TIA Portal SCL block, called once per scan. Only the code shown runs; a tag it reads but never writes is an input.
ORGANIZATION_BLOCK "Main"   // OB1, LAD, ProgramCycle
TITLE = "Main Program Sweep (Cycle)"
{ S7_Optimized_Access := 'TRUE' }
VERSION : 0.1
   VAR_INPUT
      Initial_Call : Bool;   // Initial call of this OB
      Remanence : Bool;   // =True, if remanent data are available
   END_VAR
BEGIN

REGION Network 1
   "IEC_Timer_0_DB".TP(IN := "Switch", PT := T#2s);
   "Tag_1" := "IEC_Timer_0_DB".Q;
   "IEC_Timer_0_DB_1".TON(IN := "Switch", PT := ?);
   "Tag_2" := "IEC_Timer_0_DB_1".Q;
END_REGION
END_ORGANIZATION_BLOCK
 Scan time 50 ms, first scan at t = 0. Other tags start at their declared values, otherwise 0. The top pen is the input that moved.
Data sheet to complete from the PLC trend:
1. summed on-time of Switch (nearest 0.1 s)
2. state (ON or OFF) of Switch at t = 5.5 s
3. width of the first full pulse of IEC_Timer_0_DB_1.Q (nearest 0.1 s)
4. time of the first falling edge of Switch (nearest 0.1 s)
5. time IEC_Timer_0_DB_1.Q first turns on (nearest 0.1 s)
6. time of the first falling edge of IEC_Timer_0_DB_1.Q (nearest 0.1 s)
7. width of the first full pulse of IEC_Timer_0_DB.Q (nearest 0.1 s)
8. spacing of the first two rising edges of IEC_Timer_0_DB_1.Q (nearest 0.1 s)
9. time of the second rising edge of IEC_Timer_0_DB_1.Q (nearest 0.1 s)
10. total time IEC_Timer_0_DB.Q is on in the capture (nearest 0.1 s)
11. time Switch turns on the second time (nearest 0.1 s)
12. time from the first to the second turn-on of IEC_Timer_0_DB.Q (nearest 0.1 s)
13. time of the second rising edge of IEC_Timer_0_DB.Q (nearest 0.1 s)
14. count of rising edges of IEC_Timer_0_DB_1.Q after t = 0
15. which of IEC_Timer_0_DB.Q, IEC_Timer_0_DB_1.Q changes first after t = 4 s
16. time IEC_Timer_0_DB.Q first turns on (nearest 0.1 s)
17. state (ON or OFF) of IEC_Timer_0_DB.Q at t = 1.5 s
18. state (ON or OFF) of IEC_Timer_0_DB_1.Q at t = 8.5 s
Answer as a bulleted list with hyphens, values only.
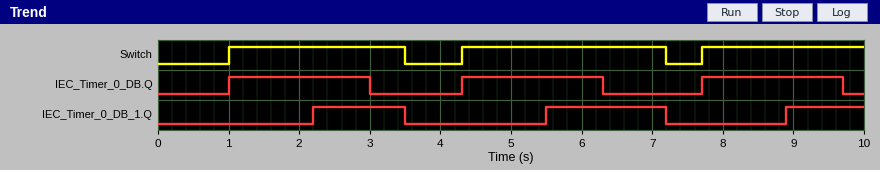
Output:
- 7.7 s
- ON
- 1.3 s
- 3.5 s
- 2.2 s
- 3.5 s
- 2.0 s
- 3.3 s
- 5.5 s
- 6.0 s
- 4.3 s
- 3.3 s
- 4.3 s
- 3
- IEC_Timer_0_DB.Q
- 1.0 s
- ON
- OFF
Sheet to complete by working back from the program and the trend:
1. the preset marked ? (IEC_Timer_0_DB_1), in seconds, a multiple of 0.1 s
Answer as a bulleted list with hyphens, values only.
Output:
- 1.2 s
